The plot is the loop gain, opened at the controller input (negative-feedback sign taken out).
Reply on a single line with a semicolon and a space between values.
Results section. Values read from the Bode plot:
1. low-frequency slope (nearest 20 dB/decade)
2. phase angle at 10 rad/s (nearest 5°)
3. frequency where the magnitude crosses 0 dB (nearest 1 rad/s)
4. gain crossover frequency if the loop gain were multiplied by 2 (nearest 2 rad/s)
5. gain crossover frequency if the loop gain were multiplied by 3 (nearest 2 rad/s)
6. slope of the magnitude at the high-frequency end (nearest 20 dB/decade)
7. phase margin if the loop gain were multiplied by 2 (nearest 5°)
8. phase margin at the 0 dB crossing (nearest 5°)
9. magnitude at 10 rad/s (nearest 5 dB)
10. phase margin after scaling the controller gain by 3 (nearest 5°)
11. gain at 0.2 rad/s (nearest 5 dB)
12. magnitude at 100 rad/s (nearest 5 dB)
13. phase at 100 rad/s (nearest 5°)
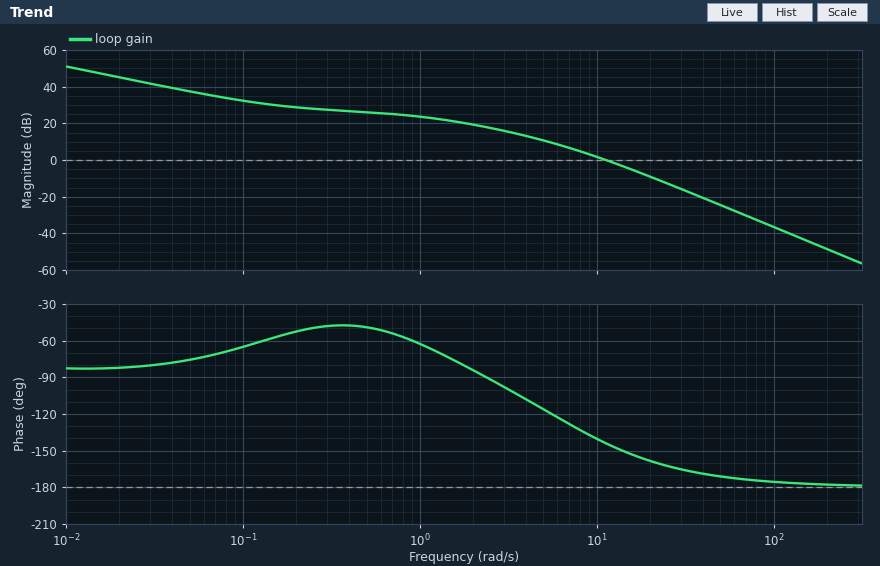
-20 dB/decade; -140°; 11 rad/s; 16 rad/s; 20 rad/s; -40 dB/decade; 25°; 35°; 0 dB; 20°; 30 dB; -35 dB; -175°
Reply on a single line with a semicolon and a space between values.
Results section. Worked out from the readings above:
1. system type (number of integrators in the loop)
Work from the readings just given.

1
